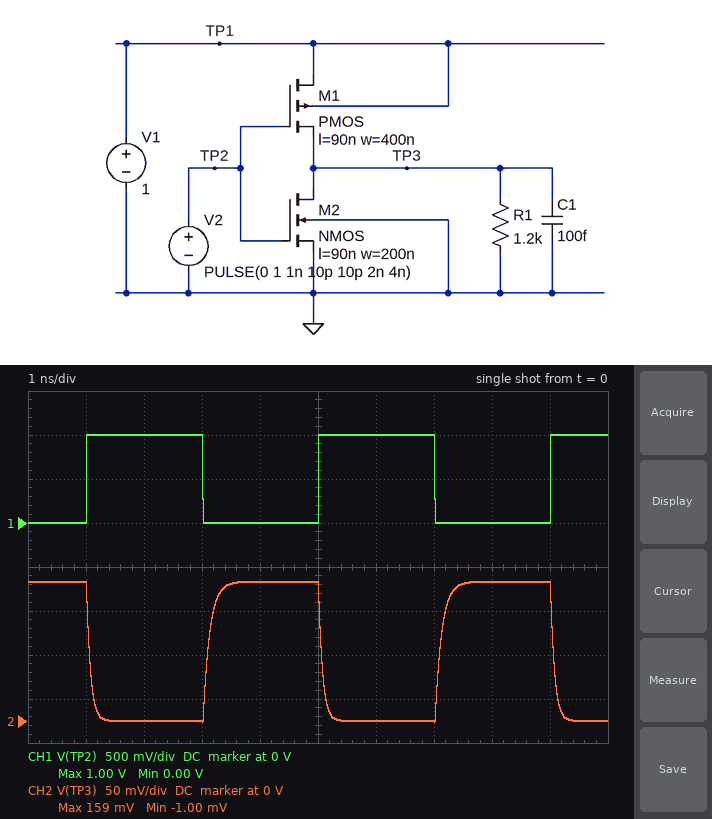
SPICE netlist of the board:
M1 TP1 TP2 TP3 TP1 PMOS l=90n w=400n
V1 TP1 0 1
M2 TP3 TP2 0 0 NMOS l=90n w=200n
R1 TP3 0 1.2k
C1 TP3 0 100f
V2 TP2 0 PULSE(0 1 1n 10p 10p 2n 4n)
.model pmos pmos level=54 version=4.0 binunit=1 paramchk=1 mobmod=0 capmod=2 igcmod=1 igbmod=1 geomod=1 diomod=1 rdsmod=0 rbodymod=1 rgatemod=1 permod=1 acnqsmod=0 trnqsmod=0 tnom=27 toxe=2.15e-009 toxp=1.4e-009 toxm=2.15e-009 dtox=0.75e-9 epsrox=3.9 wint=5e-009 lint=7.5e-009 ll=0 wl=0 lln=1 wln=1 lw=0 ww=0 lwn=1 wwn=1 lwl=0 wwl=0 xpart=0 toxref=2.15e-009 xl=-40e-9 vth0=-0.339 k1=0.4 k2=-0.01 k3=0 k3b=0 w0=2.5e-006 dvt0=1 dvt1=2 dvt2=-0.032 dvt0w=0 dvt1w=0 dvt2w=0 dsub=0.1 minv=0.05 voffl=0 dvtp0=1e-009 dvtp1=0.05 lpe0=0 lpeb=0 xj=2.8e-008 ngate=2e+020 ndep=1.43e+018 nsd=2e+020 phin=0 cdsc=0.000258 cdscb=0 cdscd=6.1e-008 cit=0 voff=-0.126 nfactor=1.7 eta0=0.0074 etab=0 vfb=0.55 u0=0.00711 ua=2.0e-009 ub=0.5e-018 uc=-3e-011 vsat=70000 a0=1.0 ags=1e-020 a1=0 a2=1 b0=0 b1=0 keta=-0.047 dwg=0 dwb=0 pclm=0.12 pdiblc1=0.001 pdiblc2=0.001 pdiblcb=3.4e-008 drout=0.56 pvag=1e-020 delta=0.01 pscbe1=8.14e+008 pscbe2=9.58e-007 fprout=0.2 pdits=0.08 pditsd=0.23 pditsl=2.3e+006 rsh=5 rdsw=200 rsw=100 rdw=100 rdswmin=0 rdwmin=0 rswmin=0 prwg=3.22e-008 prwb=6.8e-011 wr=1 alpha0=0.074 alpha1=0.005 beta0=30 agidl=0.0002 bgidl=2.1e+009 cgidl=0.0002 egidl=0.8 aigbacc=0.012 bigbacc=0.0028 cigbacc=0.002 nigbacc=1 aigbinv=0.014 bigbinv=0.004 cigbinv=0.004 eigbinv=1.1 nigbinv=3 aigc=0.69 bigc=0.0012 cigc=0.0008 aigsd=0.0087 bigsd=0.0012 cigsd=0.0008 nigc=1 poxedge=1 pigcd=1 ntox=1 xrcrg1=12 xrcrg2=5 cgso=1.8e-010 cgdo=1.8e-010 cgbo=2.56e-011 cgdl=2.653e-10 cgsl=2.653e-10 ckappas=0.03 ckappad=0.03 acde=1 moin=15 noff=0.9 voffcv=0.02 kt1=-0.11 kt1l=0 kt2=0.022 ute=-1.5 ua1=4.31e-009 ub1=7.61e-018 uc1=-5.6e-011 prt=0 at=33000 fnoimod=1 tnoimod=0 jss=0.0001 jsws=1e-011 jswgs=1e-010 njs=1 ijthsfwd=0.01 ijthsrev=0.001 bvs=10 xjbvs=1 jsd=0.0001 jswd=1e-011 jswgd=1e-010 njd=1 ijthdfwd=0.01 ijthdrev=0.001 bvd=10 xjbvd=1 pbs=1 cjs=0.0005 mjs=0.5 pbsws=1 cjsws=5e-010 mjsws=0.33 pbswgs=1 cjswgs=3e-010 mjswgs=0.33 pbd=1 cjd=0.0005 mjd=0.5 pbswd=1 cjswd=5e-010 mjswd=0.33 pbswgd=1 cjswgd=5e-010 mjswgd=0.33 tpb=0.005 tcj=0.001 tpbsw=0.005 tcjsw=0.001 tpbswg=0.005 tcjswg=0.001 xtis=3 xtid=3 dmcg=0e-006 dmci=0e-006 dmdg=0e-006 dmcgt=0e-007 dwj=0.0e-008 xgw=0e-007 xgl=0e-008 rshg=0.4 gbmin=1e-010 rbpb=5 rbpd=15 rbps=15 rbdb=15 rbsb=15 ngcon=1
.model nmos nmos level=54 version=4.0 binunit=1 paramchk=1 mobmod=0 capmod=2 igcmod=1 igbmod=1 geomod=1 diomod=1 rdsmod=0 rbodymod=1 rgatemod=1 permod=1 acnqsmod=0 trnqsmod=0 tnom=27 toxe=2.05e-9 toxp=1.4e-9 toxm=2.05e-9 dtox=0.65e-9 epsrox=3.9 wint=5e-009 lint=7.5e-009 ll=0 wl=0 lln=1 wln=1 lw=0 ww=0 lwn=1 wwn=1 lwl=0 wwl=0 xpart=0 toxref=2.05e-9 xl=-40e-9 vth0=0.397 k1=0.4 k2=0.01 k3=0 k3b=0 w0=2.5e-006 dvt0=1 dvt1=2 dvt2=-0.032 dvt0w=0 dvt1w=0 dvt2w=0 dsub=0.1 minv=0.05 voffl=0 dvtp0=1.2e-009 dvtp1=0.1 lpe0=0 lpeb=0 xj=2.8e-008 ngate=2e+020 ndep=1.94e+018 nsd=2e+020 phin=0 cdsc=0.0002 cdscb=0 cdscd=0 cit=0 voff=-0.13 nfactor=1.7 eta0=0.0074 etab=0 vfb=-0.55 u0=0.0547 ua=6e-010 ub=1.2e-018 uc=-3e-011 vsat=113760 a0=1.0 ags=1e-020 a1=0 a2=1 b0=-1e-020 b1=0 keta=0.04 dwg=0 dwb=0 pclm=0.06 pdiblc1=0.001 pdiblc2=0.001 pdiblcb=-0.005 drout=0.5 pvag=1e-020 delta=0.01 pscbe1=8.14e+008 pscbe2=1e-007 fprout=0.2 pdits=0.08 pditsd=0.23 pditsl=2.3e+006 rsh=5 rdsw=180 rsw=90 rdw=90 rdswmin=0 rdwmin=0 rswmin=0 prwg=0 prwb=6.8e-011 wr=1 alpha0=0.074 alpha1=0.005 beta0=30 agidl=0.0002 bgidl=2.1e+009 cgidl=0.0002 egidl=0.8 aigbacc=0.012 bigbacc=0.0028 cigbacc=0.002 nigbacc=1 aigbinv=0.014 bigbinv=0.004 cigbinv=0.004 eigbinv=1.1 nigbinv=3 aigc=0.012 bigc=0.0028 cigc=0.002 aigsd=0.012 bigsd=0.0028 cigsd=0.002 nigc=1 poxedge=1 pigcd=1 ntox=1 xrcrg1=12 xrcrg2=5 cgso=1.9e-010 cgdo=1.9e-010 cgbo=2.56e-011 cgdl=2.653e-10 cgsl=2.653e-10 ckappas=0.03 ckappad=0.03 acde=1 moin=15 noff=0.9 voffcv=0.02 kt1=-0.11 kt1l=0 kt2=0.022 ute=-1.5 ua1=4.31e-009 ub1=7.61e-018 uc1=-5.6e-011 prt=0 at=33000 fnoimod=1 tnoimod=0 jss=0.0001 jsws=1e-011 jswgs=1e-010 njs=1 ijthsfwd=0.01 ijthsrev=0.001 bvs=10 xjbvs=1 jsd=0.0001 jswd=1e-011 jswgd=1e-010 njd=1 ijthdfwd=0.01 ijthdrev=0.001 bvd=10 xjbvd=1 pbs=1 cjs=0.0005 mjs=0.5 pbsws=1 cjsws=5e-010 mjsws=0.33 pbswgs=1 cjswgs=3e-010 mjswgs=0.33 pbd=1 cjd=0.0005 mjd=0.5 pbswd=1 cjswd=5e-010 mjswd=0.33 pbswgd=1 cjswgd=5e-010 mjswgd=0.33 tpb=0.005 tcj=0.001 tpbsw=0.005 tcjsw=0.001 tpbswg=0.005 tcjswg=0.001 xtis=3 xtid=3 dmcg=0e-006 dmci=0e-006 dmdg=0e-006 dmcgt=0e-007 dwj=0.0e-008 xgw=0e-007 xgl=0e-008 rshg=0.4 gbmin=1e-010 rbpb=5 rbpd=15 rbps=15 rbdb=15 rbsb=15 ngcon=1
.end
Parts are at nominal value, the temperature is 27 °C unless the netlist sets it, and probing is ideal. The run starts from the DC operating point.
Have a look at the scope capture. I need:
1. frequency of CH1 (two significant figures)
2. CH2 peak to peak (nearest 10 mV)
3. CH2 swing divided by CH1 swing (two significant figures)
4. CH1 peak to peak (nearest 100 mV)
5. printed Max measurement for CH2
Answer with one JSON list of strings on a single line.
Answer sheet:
["250 MHz", "160 mV", "0.16", "1.0 V", "159 mV"]
